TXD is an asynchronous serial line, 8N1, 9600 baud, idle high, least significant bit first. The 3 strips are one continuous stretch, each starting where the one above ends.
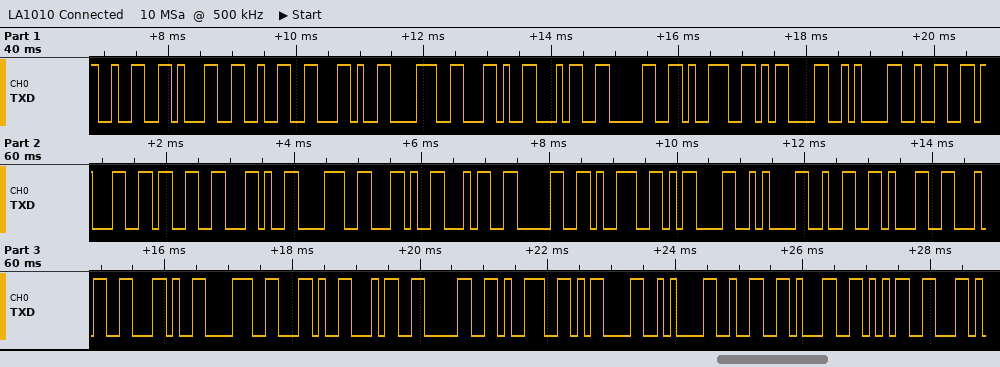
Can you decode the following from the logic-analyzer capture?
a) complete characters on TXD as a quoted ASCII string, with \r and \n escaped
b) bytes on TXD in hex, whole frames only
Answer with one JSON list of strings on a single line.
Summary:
["\"212,8,409\\r\\n213,8,409\\r\\n214,8,409\\r\\n215\"", "32 31 32 2C 38 2C 34 30 39 0D 0A 32 31 33 2C 38 2C 34 30 39 0D 0A 32 31 34 2C 38 2C 34 30 39 0D 0A 32 31 35"]
